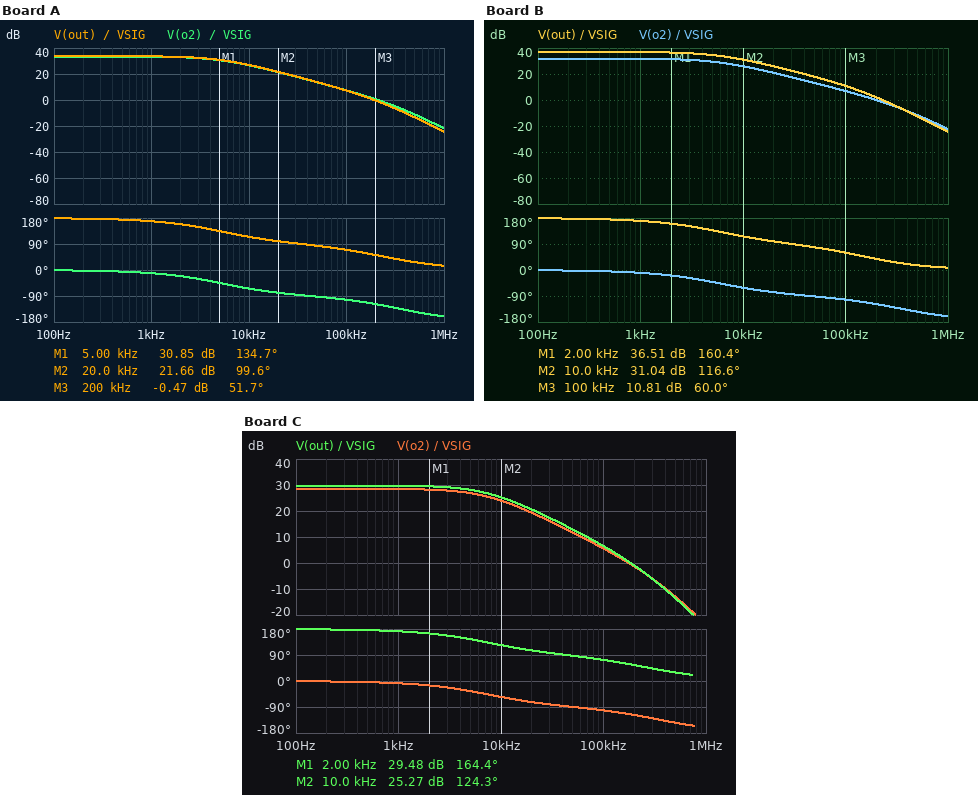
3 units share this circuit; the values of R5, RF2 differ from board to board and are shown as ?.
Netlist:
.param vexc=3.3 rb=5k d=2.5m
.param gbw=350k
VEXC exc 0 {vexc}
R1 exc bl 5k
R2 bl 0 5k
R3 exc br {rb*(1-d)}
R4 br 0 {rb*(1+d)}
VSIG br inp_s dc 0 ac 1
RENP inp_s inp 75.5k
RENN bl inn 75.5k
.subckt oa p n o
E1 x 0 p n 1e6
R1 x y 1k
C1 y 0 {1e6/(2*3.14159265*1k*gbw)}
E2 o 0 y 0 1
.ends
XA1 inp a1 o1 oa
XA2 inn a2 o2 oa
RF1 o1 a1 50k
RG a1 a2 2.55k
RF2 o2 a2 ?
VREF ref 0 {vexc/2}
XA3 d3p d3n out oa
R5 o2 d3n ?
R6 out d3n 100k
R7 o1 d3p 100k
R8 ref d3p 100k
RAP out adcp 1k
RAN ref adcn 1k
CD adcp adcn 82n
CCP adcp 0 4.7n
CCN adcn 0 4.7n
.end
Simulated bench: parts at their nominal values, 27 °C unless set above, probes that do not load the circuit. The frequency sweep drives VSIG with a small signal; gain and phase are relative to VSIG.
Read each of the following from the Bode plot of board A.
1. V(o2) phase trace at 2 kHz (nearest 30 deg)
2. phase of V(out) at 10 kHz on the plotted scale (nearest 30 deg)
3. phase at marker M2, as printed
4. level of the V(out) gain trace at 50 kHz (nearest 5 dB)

-30 deg
120 deg
99.6 deg
15 dB
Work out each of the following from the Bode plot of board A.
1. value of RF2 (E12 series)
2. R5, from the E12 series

120 kΩ
150 kΩ
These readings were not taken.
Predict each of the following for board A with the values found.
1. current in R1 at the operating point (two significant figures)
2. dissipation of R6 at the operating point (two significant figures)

330 µA
250 nW
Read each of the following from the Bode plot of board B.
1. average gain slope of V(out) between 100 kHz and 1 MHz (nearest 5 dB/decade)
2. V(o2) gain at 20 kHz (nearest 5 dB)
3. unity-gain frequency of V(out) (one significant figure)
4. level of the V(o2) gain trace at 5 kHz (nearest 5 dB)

-35 dB/decade
20 dB
200 kHz
30 dB
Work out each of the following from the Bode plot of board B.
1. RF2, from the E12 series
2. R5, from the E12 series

100 kΩ
82 kΩ
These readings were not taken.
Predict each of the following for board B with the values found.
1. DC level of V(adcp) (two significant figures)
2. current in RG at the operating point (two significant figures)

1.9 V
1.6 µA
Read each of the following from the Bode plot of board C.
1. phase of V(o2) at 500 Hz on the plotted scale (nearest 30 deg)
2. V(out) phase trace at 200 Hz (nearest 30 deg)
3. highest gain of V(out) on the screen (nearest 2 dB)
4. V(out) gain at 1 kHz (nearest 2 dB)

0 deg
180 deg
30 dB
30 dB
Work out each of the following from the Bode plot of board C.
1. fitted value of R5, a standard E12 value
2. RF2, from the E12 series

180 kΩ
68 kΩ
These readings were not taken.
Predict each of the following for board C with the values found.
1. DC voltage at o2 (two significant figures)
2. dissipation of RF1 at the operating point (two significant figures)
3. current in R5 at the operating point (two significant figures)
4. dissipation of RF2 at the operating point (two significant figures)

1.5 V
130 nW
850 nA
180 nW
